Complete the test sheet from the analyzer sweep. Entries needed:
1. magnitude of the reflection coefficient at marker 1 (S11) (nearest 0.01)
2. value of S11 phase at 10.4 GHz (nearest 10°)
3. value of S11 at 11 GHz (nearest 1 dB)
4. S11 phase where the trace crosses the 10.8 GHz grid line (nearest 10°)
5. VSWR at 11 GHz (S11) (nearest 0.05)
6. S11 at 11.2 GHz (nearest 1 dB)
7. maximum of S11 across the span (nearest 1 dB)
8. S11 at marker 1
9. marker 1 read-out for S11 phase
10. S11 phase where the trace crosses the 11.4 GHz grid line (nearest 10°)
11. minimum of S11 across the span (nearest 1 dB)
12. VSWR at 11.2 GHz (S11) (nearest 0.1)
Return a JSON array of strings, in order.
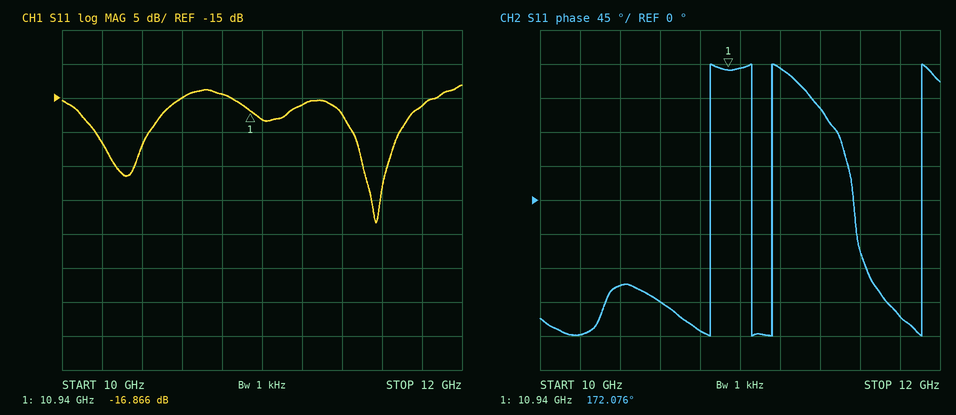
["0.14", "-110°", "-18 dB", "-170°", "1.30", "-16 dB", "-13 dB", "-16.866 dB", "172.076°", "120°", "-33 dB", "1.4"]
